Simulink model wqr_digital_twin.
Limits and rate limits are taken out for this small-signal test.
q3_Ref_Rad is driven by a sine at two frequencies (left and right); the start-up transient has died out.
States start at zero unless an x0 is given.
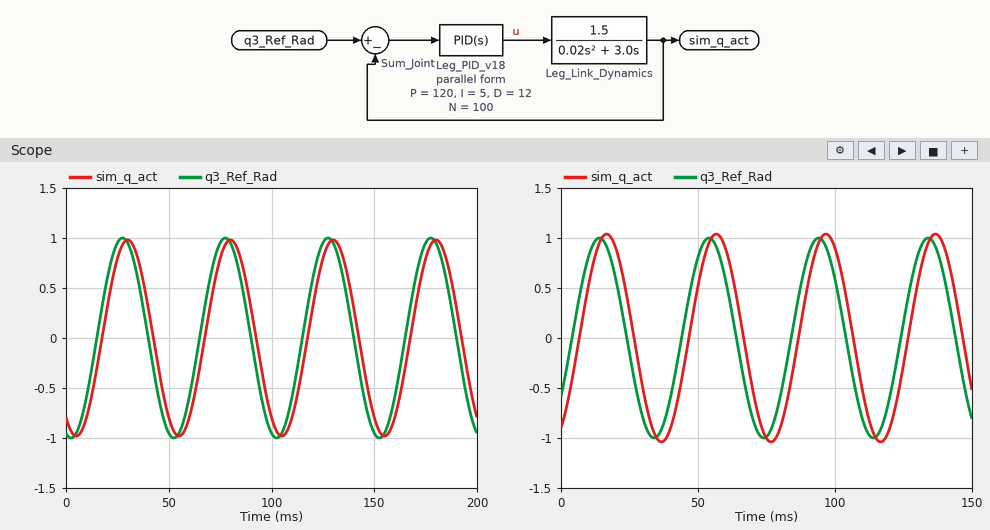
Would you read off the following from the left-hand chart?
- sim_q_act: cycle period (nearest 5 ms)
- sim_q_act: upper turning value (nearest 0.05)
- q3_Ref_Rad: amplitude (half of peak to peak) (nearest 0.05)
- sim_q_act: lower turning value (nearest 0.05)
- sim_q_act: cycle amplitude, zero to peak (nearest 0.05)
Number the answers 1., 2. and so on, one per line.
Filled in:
1. 50 ms
2. 1.00
3. 1.00
4. -1.00
5. 1.00
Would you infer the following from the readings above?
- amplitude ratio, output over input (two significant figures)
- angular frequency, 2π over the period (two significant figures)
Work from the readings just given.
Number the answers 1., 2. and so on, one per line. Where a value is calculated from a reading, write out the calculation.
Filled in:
1. 1 / 1 = 1.0
2. 2π / 50 = 0.13 rad/ms
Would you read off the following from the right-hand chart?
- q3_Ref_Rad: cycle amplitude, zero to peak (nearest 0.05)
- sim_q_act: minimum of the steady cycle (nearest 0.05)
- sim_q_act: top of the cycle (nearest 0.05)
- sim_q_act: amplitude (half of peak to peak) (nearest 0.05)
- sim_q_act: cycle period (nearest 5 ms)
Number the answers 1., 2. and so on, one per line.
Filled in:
1. 1.00
2. -1.05
3. 1.05
4. 1.05
5. 40 ms
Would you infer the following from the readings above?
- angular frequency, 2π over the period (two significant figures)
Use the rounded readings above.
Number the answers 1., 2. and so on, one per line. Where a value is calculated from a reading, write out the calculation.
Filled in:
1. 2π / 40 = 0.16 rad/ms
